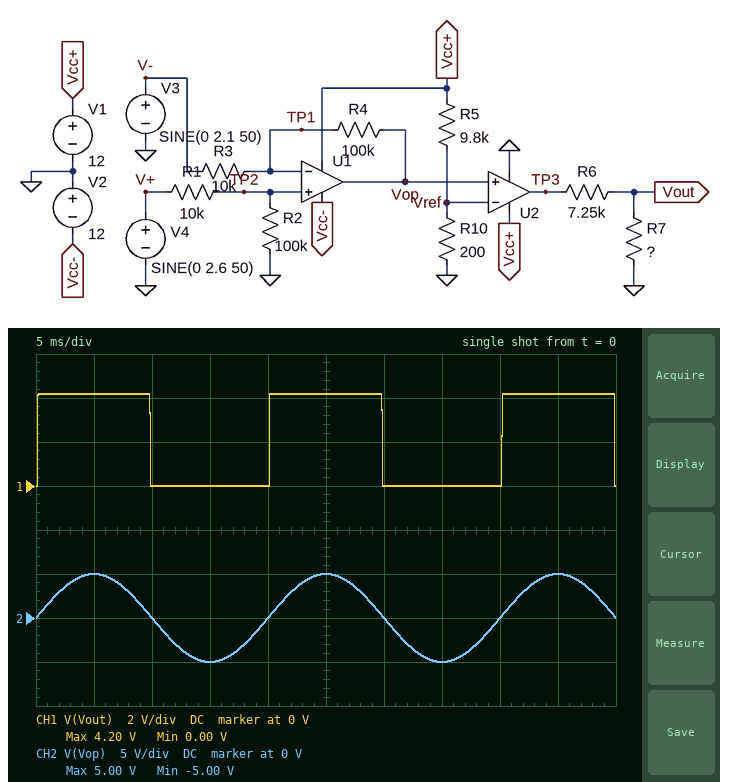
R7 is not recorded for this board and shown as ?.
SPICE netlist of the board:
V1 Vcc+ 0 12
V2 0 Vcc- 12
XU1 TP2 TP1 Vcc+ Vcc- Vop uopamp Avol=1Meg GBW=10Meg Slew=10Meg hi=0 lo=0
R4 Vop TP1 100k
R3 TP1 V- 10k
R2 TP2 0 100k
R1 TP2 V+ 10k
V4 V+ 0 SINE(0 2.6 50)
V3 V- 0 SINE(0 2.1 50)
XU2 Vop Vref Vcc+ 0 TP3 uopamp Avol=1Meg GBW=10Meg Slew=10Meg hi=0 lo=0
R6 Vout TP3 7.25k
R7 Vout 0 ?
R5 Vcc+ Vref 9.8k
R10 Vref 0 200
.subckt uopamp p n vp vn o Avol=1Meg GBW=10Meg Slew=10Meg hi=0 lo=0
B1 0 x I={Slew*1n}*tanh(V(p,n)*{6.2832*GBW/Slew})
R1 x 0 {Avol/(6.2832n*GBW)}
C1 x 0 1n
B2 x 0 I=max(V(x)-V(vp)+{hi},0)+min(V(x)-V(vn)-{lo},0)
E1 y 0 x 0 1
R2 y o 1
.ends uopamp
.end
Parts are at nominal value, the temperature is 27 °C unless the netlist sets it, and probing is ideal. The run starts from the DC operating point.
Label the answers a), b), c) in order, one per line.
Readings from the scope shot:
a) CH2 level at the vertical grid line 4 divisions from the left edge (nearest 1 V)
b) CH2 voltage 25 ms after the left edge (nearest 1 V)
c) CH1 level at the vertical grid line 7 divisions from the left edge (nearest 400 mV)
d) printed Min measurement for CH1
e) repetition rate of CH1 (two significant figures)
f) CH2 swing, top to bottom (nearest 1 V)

a) 0 V
b) 5 V
c) 0 V
d) 0.00 V
e) 50 Hz
f) 10 V
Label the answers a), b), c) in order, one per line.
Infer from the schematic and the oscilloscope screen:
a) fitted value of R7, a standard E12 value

a) 3.9 kΩ
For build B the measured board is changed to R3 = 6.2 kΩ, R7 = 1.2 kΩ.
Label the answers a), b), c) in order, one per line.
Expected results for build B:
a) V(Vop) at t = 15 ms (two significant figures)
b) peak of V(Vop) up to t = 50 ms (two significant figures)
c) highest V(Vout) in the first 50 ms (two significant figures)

a) -6.6 V
b) 6.6 V
c) 1.7 V
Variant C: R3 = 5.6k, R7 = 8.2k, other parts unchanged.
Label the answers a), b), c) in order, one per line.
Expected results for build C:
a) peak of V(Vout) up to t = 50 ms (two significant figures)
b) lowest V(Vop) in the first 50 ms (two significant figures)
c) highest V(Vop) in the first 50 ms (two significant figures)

a) 6.4 V
b) -7.1 V
c) 7.1 V
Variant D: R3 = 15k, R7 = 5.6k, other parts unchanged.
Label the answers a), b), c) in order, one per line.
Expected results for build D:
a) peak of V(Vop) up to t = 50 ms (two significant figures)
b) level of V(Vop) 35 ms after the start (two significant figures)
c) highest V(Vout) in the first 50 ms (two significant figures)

a) 4.1 V
b) -4.1 V
c) 5.2 V
